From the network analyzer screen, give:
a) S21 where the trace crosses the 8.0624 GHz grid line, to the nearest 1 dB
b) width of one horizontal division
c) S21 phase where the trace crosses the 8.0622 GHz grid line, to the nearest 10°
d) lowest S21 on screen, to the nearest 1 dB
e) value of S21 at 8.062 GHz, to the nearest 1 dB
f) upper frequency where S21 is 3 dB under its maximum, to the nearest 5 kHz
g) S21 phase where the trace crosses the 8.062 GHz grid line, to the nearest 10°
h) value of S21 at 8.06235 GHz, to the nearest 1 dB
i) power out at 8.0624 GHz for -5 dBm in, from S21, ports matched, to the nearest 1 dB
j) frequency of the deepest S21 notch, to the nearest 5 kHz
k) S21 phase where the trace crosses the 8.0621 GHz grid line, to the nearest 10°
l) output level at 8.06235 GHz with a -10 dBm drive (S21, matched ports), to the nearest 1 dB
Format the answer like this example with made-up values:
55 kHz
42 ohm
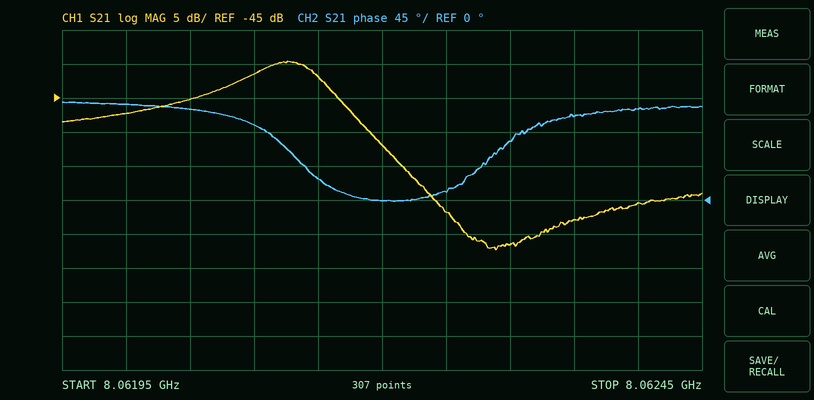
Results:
-60 dB
50 kHz
0°
-67 dB
-47 dB
8.062155 GHz
130°
-63 dB
-65 dBm
8.062290 GHz
100°
-73 dBm
